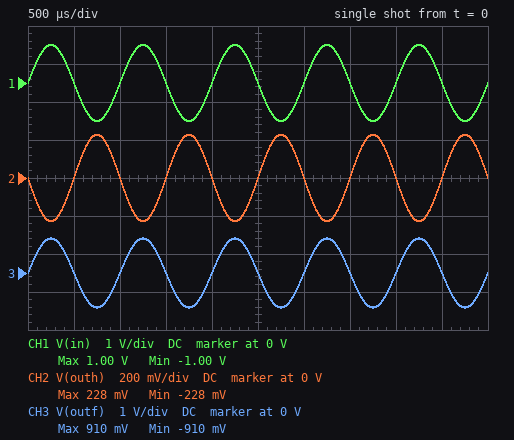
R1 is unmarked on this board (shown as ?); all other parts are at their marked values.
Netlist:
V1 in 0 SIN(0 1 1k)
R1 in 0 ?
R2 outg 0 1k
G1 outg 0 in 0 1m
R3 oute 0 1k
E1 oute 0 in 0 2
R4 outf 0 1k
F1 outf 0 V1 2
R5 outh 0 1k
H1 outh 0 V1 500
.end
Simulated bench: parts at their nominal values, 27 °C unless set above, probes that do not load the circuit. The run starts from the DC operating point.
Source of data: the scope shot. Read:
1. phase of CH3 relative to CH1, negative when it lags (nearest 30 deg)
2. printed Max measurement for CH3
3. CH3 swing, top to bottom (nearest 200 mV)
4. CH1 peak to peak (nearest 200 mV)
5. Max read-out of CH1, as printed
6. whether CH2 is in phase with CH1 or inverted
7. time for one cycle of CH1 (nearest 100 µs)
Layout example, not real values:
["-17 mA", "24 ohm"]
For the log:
["0 deg", "910 mV", "1.8 V", "2.0 V", "1.00 V", "inverted", "1.0 ms"]
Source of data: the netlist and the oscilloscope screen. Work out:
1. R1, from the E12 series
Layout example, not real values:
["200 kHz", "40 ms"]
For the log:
["2.2 kΩ"]
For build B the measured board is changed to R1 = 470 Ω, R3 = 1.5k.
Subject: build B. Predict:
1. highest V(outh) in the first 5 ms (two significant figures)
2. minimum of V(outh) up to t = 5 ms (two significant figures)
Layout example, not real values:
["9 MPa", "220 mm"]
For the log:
["1.1 V", "-1.1 V"]
